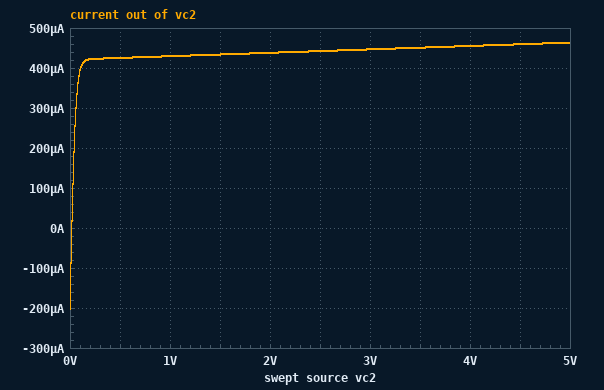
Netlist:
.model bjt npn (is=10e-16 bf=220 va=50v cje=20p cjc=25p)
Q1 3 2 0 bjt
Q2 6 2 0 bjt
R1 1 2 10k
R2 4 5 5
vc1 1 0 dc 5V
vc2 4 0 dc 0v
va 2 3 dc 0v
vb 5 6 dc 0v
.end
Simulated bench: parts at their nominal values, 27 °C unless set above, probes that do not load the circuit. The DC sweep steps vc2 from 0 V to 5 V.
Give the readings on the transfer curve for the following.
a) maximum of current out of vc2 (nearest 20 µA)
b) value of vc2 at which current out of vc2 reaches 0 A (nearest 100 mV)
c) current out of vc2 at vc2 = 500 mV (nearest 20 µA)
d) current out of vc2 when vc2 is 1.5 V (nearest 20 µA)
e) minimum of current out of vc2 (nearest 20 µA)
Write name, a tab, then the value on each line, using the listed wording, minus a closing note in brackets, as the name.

maximum of current out of vc2	460 µA
value of vc2 at which current out of vc2 reaches 0 A	0 V
current out of vc2 at vc2 = 500 mV	420 µA
current out of vc2 when vc2 is 1.5 V	440 µA
minimum of current out of vc2	-200 µA
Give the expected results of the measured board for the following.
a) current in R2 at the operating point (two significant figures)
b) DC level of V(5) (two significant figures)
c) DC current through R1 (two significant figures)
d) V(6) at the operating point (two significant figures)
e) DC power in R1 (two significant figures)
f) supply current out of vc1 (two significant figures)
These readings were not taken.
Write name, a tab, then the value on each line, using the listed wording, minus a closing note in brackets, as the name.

current in R2 at the operating point	200 µA
DC level of V(5)	1.0 mV
DC current through R1	430 µA
V(6) at the operating point	1.0 mV
DC power in R1	1.9 mW
supply current out of vc1	430 µA
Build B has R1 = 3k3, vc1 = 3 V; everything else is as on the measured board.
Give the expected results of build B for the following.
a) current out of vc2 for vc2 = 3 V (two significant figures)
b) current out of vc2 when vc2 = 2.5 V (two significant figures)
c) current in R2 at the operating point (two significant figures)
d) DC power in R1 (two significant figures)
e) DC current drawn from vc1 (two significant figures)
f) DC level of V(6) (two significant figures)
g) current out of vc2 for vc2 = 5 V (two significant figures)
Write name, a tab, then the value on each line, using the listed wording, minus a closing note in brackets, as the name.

current out of vc2 for vc2 = 3 V	720 µA
current out of vc2 when vc2 = 2.5 V	710 µA
current in R2 at the operating point	320 µA
DC power in R1	1.6 mW
DC current drawn from vc1	700 µA
DC level of V(6)	1.6 mV
current out of vc2 for vc2 = 5 V	750 µA
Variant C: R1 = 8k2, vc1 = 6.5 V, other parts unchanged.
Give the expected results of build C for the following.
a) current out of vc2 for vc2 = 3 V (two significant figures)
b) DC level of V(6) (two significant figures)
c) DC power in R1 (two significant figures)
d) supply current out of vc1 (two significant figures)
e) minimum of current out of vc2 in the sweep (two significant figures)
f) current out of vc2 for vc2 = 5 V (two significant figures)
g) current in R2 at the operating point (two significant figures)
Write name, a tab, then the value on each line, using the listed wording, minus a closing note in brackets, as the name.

current out of vc2 for vc2 = 3 V	730 µA
DC level of V(6)	1.6 mV
DC power in R1	4.1 mW
supply current out of vc1	710 µA
minimum of current out of vc2 in the sweep	-320 µA
current out of vc2 for vc2 = 5 V	760 µA
current in R2 at the operating point	320 µA
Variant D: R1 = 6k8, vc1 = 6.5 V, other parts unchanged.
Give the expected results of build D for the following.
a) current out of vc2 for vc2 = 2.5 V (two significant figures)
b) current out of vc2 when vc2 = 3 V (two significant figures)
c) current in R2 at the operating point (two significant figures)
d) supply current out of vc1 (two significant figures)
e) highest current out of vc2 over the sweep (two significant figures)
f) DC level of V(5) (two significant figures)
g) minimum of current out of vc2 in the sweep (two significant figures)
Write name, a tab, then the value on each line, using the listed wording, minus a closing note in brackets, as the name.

current out of vc2 for vc2 = 2.5 V	870 µA
current out of vc2 when vc2 = 3 V	880 µA
current in R2 at the operating point	380 µA
supply current out of vc1	850 µA
highest current out of vc2 over the sweep	920 µA
DC level of V(5)	1.9 mV
minimum of current out of vc2 in the sweep	-380 µA
